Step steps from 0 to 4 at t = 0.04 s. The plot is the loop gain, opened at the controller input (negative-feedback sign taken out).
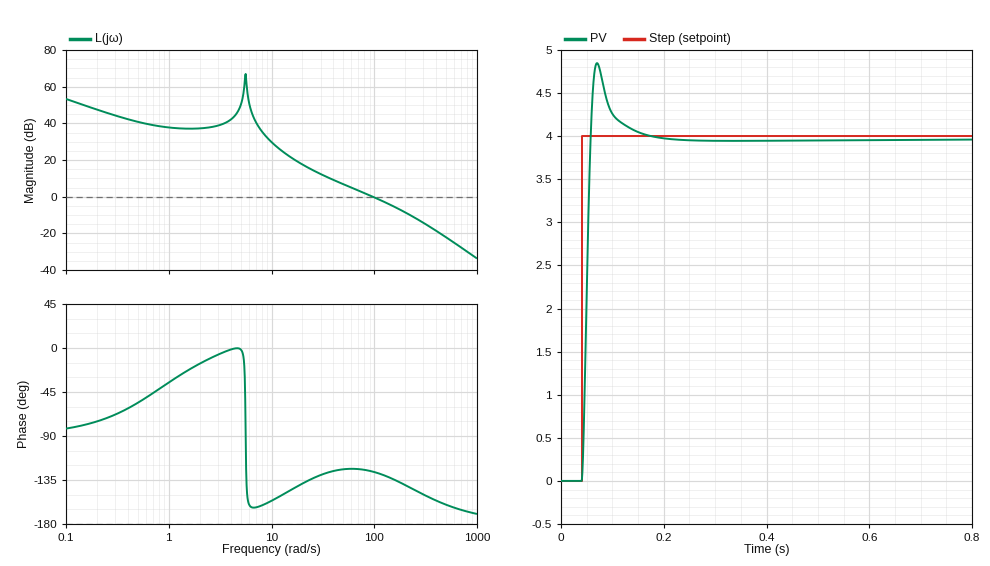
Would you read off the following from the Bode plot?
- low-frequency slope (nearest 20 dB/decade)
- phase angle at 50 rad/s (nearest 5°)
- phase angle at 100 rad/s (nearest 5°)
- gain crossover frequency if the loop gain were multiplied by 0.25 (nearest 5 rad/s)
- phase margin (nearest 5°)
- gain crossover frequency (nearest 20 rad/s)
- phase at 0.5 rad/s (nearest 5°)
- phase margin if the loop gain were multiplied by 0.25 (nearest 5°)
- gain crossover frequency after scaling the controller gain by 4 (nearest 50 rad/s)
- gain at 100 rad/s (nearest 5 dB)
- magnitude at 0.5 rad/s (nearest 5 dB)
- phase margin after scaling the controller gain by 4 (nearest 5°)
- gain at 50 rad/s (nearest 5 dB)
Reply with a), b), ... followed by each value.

a) -20 dB/decade
b) -125°
c) -125°
d) 30 rad/s
e) 55°
f) 100 rad/s
g) -55°
h) 50°
i) 250 rad/s
j) 0 dB
k) 40 dB
l) 35°
m) 5 dB
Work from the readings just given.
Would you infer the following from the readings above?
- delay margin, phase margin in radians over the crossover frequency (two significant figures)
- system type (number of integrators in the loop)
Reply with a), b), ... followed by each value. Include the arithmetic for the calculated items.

a) 55 × π / 180 / 100 = 0.0096 s
b) 1
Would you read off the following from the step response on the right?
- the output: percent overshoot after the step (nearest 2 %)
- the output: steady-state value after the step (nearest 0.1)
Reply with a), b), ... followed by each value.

a) 22 %
b) 4.0
